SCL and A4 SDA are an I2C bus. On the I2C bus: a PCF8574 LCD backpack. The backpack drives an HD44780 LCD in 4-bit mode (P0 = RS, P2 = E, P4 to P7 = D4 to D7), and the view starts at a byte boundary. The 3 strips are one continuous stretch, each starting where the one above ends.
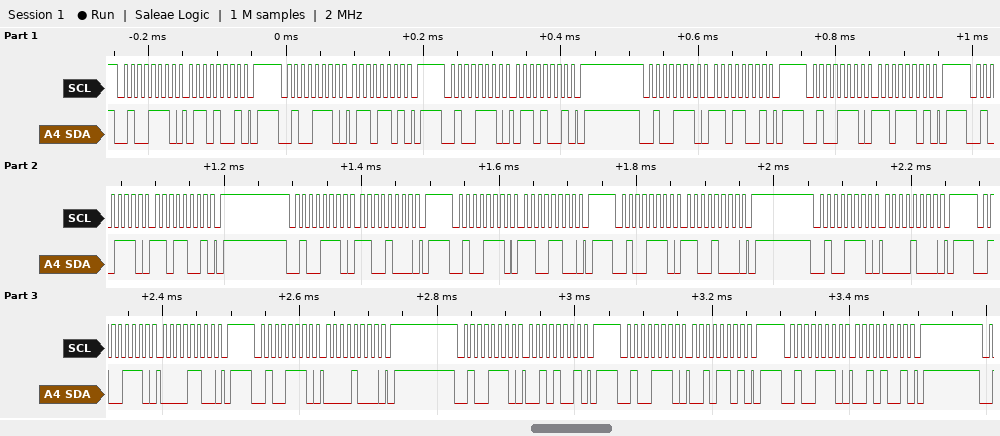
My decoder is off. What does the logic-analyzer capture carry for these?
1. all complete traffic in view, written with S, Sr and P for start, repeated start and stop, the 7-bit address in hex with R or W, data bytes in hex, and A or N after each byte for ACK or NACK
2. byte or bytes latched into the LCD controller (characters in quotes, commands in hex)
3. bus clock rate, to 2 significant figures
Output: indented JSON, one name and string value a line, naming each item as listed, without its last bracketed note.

{
  "all complete traffic in view, written with S, Sr and P for start, repeated start and stop, the 7-bit address in hex with R or W, data bytes in hex, and A or N after each byte for ACK or NACK": "S 27W A 69 A P S 27W A 6D A P S 27W A 69 A P S 27W A D9 A P S 27W A DD A P S 27W A D9 A P S 27W A C8 A P S 27W A CC A P S 27W A C8 A P S 27W A 08 A P S 27W A 0C A P S 27W A 08 A P S 27W A 29 A P S 27W A 2D A P S 27W A 29 A P",
  "byte or bytes latched into the LCD controller": "'m' 0xC0",
  "bus clock rate, to 2 significant figures": "100 kHz"
}
